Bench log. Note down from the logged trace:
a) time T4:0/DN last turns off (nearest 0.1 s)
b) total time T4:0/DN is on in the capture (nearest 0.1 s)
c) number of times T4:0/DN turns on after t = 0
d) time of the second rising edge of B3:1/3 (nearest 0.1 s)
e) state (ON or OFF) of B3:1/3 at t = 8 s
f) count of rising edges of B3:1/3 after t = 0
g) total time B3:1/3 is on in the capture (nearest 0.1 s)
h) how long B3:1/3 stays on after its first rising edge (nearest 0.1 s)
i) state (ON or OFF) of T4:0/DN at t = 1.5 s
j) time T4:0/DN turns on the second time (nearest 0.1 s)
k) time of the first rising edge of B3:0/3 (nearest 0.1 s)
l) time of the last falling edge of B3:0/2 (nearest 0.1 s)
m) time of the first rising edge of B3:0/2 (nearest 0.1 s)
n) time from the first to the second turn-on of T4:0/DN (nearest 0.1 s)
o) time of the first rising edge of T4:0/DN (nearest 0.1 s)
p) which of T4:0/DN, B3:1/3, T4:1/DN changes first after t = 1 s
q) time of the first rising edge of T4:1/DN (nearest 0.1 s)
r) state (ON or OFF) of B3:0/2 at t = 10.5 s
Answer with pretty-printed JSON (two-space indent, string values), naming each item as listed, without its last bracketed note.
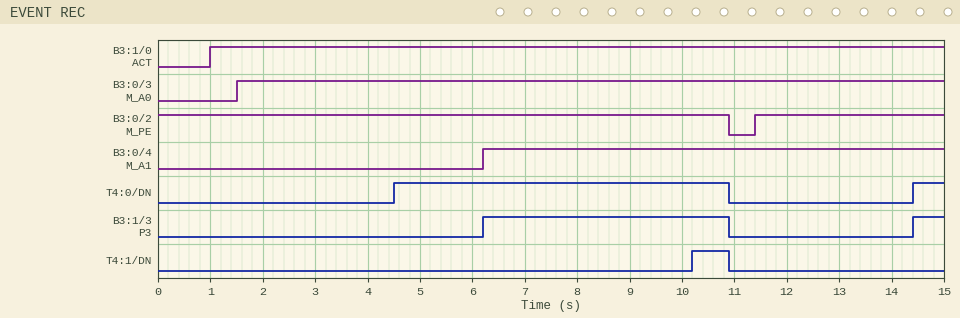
{
  "time T4:0/DN last turns off": "10.9 s",
  "total time T4:0/DN is on in the capture": "7.0 s",
  "number of times T4:0/DN turns on after t = 0": "2",
  "time of the second rising edge of B3:1/3": "14.4 s",
  "state (ON or OFF) of B3:1/3 at t = 8 s": "ON",
  "count of rising edges of B3:1/3 after t = 0": "2",
  "total time B3:1/3 is on in the capture": "5.3 s",
  "how long B3:1/3 stays on after its first rising edge": "4.7 s",
  "state (ON or OFF) of T4:0/DN at t = 1.5 s": "OFF",
  "time T4:0/DN turns on the second time": "14.4 s",
  "time of the first rising edge of B3:0/3": "1.5 s",
  "time of the last falling edge of B3:0/2": "10.9 s",
  "time of the first rising edge of B3:0/2": "11.4 s",
  "time from the first to the second turn-on of T4:0/DN": "9.9 s",
  "time of the first rising edge of T4:0/DN": "4.5 s",
  "which of T4:0/DN, B3:1/3, T4:1/DN changes first after t = 1 s": "T4:0/DN",
  "time of the first rising edge of T4:1/DN": "10.2 s",
  "state (ON or OFF) of B3:0/2 at t = 10.5 s": "ON"
}
